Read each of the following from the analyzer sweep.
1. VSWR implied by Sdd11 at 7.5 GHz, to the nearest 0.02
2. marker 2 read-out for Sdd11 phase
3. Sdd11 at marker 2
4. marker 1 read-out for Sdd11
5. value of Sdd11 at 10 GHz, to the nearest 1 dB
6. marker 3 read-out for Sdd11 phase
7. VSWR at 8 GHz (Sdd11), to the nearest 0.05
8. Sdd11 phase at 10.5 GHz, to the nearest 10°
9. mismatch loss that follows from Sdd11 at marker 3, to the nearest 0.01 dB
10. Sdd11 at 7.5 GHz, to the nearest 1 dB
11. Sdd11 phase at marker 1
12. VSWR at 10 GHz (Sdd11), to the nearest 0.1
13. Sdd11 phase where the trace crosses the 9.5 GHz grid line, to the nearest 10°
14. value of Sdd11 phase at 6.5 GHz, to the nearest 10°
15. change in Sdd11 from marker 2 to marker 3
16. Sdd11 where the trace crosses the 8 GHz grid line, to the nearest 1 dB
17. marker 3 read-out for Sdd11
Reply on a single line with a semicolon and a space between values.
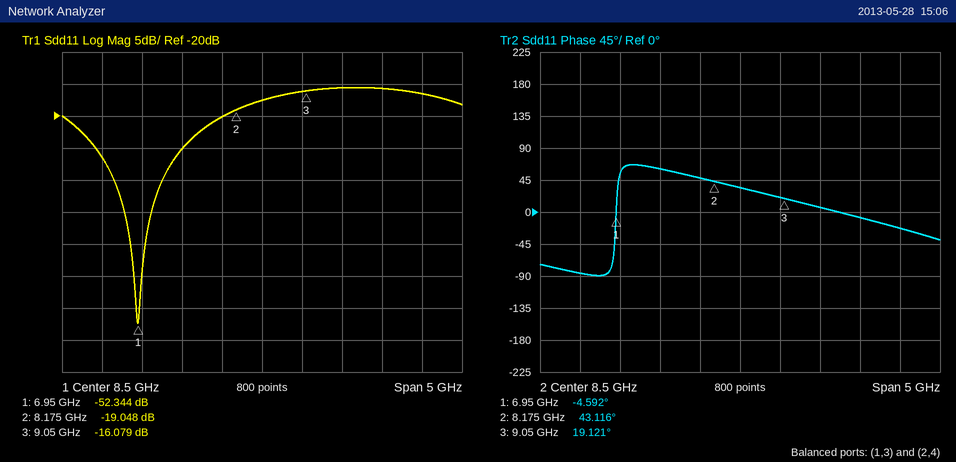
1.12; 43.116°; -19.048 dB; -52.344 dB; -16 dB; 19.121°; 1.20; -20°; 0.11 dB; -25 dB; -4.592°; 1.4; 10°; -90°; 2.969 dB; -20 dB; -16.079 dB
